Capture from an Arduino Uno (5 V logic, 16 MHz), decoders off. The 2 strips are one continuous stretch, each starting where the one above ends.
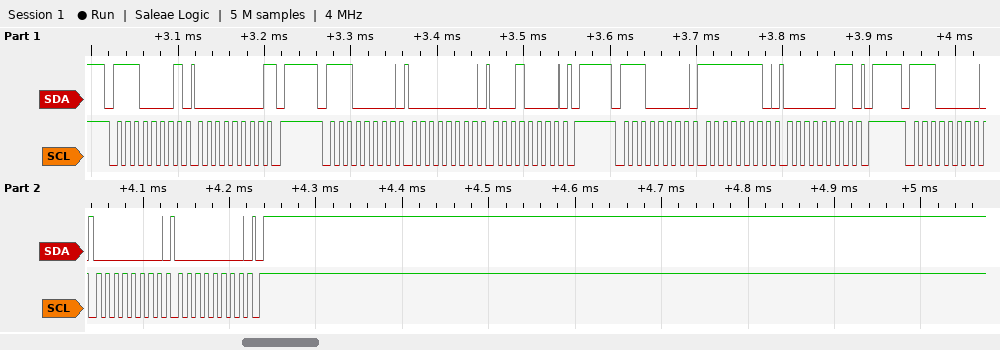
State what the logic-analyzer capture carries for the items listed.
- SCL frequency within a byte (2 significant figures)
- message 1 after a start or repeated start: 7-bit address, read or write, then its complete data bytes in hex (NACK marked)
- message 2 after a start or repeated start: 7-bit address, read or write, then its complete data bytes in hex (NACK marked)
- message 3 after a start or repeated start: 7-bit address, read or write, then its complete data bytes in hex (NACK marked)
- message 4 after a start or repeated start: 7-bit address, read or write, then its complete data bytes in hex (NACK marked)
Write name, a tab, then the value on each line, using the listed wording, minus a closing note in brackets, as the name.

SCL frequency within a byte	100 kHz
message 1 after a start or repeated start: 7-bit address, read or write, then its complete data bytes in hex	0x70 read: 00 NACK
message 2 after a start or repeated start: 7-bit address, read or write, then its complete data bytes in hex	0x70 write: 00 10
message 3 after a start or repeated start: 7-bit address, read or write, then its complete data bytes in hex	0x70 write: FE 03
message 4 after a start or repeated start: 7-bit address, read or write, then its complete data bytes in hex	0x70 write: 00 00
